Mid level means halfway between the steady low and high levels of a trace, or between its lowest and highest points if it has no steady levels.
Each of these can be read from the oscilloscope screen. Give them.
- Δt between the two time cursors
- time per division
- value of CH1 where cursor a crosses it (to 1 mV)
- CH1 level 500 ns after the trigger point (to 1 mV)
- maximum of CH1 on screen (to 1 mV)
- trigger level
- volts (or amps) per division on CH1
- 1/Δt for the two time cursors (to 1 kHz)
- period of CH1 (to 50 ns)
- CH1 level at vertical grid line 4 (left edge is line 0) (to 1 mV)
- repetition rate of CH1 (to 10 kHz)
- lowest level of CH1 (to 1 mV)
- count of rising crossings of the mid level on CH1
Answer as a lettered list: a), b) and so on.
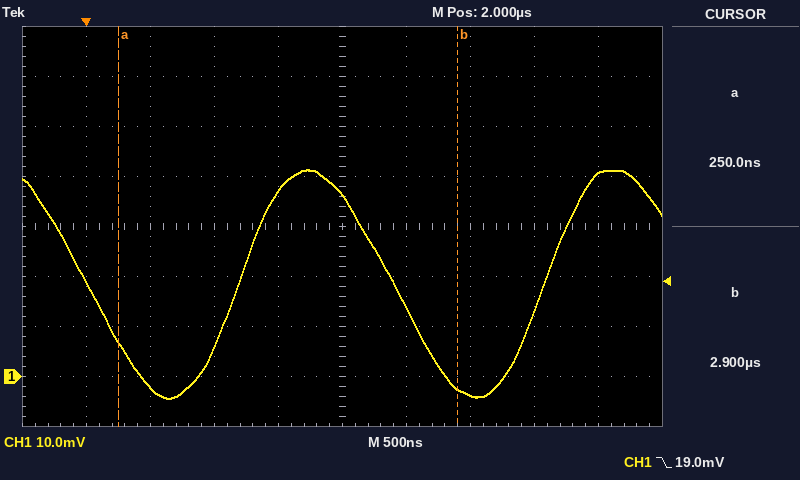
a) 2.65 µs
b) 500 ns
c) 7 mV
d) -2 mV
e) 41 mV
f) 19.0 mV
g) 10 mV
h) 377 kHz
i) 2.40 µs
j) 37 mV
k) 420 kHz
l) -4 mV
m) 2
